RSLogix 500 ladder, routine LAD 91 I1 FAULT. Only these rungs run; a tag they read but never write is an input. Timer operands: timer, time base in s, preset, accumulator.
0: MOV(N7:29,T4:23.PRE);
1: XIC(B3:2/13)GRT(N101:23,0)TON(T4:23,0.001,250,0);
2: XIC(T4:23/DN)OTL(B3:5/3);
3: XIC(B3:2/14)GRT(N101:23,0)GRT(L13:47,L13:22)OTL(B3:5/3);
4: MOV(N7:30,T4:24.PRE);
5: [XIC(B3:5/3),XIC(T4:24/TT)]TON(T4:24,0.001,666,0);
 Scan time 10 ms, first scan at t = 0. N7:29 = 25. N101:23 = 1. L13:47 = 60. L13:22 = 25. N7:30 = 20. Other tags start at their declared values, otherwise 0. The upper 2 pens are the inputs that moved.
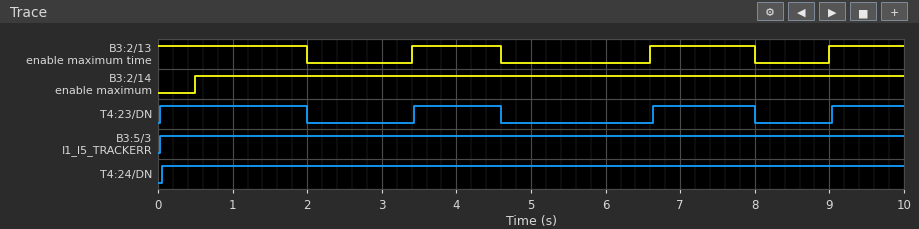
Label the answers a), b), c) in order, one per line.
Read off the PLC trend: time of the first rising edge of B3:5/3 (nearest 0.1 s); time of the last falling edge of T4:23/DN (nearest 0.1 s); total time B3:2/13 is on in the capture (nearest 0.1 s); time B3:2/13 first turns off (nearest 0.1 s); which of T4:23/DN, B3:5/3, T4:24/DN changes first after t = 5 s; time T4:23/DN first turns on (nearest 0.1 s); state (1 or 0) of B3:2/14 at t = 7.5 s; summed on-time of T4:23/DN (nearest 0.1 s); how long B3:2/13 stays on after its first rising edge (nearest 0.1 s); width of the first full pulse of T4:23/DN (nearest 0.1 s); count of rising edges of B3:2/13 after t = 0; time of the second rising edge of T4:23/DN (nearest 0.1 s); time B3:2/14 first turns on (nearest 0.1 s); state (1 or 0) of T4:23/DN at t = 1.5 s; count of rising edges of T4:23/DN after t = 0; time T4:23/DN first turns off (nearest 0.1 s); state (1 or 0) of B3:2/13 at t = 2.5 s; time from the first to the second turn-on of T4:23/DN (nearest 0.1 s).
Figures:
a) 0.0 s
b) 8.0 s
c) 5.6 s
d) 2.0 s
e) T4:23/DN
f) 0.0 s
g) 1
h) 5.5 s
i) 1.2 s
j) 2.0 s
k) 3
l) 3.4 s
m) 0.5 s
n) 1
o) 4
p) 2.0 s
q) 0
r) 3.4 s
